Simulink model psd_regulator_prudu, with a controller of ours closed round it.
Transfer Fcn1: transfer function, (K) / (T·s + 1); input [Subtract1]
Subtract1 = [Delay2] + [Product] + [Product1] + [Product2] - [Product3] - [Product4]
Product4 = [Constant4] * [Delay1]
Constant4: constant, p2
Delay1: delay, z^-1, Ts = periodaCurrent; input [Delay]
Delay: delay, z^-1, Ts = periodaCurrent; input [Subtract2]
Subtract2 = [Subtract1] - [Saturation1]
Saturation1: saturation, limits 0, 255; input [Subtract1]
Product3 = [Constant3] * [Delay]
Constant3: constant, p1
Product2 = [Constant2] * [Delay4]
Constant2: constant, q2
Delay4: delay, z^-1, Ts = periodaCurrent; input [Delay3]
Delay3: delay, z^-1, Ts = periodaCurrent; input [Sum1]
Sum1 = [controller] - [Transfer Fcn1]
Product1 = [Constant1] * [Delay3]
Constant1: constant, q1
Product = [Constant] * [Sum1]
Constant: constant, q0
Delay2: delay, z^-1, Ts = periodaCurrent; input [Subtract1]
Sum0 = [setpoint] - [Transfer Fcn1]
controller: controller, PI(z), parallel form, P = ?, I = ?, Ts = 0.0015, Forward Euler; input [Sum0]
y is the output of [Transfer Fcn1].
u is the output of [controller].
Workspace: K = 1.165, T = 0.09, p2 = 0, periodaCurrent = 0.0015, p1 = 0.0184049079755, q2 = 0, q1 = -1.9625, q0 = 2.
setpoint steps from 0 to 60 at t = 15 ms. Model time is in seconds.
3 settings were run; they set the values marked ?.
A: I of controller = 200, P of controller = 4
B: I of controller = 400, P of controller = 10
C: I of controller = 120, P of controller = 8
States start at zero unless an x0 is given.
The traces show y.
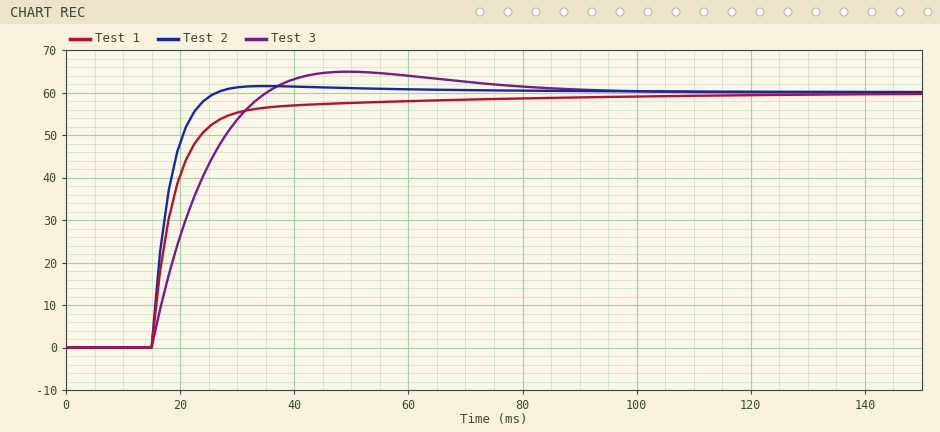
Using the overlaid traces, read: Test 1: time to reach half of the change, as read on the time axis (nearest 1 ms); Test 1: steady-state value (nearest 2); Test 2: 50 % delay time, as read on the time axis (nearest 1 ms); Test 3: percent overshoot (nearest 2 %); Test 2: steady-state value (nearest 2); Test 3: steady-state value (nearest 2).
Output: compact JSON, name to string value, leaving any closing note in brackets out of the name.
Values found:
{"Test 1: time to reach half of the change, as read on the time axis": "18 ms", "Test 1: steady-state value": "60", "Test 2: 50 % delay time, as read on the time axis": "17 ms", "Test 3: percent overshoot": "8 %", "Test 2: steady-state value": "60", "Test 3: steady-state value": "60"}
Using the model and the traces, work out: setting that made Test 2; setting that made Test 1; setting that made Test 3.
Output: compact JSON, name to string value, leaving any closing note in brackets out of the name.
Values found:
{"setting that made Test 2": "B", "setting that made Test 1": "C", "setting that made Test 3": "A"}
